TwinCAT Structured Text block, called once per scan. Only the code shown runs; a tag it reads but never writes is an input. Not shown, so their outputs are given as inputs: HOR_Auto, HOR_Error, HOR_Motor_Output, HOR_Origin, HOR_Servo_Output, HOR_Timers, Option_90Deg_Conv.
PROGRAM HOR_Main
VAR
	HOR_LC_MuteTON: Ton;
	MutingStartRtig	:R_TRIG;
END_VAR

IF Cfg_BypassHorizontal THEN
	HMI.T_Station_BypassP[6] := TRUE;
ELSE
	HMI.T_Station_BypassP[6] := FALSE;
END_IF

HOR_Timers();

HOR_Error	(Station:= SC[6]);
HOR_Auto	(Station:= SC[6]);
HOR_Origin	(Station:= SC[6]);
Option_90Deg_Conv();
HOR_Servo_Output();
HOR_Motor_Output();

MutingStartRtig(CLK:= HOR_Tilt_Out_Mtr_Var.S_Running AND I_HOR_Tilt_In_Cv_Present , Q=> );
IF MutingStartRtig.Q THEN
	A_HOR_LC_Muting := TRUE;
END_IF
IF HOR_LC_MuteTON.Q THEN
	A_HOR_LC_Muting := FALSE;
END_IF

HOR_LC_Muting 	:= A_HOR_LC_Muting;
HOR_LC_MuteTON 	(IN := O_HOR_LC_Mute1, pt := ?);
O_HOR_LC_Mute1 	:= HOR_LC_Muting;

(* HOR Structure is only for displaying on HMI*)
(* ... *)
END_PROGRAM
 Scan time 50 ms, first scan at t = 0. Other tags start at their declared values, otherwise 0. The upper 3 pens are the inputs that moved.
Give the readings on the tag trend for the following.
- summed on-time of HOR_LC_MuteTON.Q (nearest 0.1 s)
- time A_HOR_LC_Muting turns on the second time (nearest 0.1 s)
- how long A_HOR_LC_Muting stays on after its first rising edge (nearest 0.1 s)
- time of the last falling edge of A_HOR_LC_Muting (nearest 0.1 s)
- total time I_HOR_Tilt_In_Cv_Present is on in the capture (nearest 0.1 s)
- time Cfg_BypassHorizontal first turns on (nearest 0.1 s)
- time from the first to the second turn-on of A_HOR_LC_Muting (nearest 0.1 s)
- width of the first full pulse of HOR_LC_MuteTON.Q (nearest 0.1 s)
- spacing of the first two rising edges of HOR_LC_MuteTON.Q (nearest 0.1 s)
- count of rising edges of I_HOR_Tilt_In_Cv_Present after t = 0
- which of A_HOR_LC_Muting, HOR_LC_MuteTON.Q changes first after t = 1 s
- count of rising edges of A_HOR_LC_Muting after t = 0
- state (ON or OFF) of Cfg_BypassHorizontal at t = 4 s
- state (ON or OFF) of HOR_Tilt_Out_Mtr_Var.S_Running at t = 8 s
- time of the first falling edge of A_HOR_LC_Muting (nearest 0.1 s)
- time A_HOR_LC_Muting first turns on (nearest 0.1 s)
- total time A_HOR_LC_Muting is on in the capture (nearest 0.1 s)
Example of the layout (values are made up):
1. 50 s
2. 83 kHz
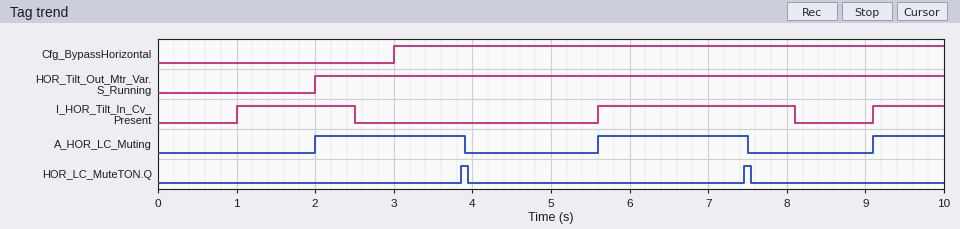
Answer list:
1. 0.2 s
2. 5.6 s
3. 1.9 s
4. 7.5 s
5. 4.9 s
6. 3.0 s
7. 3.6 s
8. 0.1 s
9. 3.6 s
10. 3
11. A_HOR_LC_Muting
12. 3
13. ON
14. ON
15. 3.9 s
16. 2.0 s
17. 4.7 s
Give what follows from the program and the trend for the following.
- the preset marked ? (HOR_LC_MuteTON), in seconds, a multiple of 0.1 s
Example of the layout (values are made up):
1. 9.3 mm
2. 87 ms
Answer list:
1. 1.8 s
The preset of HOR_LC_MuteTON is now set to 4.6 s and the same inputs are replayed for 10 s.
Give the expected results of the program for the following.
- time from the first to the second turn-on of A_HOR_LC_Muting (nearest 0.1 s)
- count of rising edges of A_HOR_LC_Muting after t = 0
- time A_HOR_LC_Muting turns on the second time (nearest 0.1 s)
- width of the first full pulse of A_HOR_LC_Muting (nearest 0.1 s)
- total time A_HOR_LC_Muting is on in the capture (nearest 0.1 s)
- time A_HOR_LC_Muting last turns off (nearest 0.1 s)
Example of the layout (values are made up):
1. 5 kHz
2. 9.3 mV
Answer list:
1. 7.1 s
2. 2
3. 9.1 s
4. 4.7 s
5. 5.6 s
6. 6.7 s
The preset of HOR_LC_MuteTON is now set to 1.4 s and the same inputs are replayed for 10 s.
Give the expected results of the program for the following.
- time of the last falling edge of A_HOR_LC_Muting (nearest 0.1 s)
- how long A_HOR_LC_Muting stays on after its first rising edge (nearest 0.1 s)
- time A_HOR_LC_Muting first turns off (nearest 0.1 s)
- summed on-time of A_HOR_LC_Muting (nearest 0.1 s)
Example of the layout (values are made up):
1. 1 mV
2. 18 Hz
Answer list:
1. 7.1 s
2. 1.5 s
3. 3.5 s
4. 3.9 s
